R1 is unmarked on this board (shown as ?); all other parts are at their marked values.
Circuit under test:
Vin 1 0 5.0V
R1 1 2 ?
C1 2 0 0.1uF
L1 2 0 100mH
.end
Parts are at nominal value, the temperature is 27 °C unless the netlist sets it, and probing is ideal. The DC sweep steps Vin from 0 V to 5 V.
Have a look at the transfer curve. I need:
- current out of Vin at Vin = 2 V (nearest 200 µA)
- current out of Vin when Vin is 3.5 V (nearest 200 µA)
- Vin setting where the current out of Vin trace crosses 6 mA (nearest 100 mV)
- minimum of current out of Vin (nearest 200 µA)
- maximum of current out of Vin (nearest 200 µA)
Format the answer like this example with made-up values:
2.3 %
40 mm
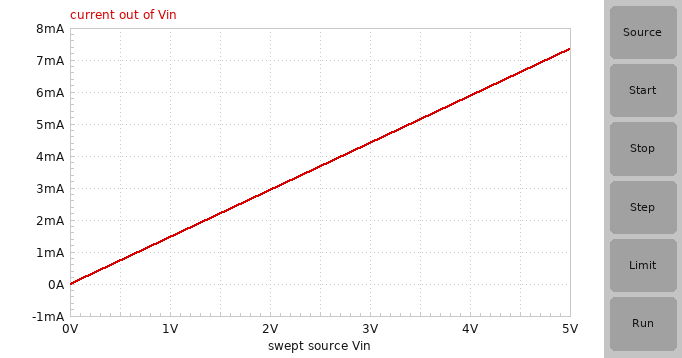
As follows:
3.0 mA
5.2 mA
4.1 V
0 A
7.4 mA
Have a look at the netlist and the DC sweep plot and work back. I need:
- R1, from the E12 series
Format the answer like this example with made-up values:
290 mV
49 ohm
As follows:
680 Ω
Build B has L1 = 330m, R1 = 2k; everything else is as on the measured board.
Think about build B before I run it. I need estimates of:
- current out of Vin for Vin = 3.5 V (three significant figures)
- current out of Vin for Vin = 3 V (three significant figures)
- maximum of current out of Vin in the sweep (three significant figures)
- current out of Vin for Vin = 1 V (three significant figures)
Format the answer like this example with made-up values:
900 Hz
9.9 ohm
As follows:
1.75 mA
1.50 mA
2.50 mA
500 µA
